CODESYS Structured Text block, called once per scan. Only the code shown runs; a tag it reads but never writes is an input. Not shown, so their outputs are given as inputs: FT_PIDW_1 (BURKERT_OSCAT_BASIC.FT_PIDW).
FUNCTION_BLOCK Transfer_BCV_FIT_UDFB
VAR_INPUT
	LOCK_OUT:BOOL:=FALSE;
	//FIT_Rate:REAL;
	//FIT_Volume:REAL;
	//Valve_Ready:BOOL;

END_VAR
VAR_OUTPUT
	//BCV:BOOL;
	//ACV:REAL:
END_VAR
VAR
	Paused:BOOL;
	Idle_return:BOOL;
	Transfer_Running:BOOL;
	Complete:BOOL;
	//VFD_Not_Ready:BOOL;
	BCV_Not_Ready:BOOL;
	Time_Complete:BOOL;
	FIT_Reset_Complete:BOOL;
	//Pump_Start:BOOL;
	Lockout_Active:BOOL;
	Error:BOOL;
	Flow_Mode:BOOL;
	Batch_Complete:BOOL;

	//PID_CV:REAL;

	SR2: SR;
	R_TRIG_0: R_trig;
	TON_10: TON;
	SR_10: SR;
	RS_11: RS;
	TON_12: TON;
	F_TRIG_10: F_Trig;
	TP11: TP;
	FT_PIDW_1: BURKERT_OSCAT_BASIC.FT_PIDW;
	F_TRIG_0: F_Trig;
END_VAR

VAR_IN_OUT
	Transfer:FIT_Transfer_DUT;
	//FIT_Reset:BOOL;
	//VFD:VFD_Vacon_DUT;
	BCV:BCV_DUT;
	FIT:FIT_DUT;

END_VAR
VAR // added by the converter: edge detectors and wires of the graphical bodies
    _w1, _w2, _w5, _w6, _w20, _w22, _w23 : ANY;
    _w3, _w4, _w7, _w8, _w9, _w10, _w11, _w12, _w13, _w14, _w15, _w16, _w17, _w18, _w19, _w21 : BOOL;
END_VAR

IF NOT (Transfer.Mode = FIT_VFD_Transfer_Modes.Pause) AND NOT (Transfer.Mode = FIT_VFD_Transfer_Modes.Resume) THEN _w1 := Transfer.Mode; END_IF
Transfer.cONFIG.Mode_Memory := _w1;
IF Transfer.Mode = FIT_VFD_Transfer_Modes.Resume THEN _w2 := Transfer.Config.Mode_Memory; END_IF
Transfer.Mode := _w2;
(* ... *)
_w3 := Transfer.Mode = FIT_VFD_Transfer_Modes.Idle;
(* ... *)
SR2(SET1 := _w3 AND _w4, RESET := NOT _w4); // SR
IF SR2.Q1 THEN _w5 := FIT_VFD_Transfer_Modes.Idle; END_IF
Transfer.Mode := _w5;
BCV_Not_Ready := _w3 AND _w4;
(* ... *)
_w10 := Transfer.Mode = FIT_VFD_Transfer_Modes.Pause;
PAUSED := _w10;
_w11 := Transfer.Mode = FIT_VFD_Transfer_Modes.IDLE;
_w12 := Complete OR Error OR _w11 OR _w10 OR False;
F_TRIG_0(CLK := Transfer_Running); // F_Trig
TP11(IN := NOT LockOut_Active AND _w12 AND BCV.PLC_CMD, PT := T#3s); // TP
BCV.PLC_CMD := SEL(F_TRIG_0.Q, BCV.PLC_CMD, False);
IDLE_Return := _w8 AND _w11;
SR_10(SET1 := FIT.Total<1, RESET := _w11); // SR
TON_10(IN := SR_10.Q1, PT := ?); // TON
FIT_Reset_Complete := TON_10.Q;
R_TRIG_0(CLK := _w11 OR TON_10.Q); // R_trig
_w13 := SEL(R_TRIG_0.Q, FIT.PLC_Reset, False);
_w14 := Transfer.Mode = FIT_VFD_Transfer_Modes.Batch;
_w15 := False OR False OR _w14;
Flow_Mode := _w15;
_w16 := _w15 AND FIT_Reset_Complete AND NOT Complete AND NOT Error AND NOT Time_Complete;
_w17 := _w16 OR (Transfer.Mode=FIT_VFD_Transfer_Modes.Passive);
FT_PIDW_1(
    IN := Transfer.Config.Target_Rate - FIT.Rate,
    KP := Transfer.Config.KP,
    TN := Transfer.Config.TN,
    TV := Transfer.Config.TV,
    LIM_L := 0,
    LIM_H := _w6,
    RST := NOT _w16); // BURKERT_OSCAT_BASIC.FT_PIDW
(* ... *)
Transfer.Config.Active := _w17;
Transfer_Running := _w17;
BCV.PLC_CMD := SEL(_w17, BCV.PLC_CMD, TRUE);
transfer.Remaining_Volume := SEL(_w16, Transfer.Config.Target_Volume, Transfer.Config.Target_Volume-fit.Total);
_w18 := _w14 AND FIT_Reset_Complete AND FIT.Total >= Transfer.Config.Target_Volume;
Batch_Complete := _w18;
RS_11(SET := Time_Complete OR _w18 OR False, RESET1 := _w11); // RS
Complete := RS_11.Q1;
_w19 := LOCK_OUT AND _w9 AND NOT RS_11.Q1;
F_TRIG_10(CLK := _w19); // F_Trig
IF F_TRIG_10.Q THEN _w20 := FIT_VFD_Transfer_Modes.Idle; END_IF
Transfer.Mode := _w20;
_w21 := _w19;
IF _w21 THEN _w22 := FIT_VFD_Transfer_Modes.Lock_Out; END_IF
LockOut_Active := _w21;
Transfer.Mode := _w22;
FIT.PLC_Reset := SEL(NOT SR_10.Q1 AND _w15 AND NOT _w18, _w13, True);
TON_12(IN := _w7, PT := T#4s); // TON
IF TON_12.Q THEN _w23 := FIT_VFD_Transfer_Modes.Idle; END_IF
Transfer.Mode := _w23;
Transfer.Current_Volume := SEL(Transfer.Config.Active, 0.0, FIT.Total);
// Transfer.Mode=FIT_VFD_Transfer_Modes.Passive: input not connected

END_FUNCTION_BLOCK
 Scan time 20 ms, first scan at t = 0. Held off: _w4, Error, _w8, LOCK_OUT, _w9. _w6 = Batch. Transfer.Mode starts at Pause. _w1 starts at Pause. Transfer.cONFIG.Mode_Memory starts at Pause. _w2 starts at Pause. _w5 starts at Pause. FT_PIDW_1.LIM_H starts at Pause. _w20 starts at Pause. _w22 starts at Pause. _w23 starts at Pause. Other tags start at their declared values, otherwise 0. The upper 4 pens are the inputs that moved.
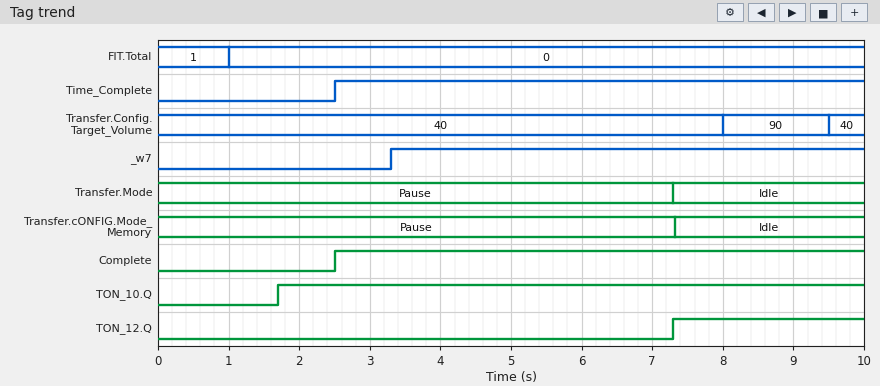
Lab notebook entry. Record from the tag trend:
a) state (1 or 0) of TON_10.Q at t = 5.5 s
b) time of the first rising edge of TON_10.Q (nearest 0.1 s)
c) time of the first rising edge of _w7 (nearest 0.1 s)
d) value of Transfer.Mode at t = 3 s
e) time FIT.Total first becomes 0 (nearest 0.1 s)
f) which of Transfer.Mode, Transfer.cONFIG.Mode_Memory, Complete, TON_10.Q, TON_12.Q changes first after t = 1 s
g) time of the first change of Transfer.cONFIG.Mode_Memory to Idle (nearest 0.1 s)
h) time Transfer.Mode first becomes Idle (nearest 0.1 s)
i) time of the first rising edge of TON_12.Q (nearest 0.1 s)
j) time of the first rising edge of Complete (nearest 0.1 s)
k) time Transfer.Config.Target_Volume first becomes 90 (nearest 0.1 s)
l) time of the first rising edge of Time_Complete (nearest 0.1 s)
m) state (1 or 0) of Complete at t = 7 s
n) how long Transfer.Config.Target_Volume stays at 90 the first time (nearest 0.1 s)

1
1.7 s
3.3 s
Pause
1.0 s
TON_10.Q
7.3 s
7.3 s
7.3 s
2.5 s
8.0 s
2.5 s
1
1.5 s
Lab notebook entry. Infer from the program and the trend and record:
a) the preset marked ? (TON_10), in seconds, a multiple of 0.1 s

0.7 s
